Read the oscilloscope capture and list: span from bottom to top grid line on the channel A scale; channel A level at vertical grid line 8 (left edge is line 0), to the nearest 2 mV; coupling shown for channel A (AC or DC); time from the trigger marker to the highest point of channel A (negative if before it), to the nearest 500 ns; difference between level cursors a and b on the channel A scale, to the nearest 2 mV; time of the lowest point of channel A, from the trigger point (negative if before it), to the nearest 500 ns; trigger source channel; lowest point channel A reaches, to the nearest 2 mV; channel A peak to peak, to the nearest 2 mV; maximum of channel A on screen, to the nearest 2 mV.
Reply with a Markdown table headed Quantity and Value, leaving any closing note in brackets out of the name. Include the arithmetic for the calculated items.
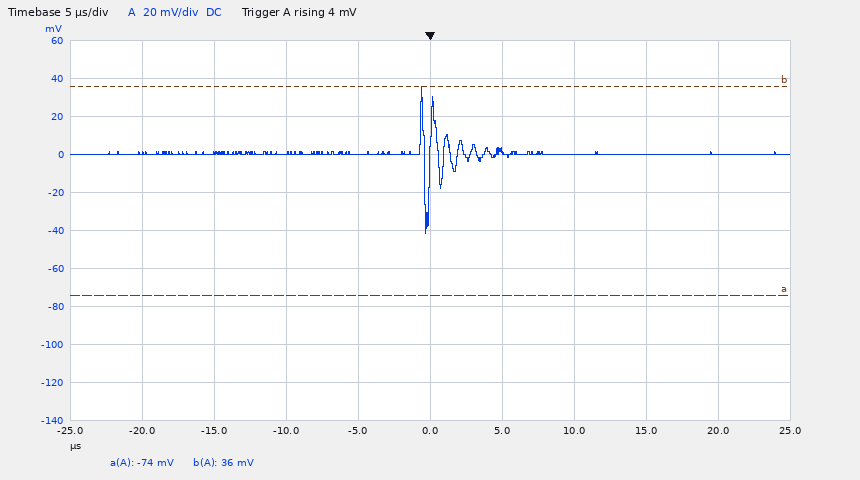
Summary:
| Quantity | Value |
|---|---|
| span from bottom to top grid line on the channel A scale | 200 mV |
| channel A level at vertical grid line 8 (left edge is line 0), to the nearest 2 mV | 0 mV |
| coupling shown for channel A | DC |
| time from the trigger marker to the highest point of channel A (negative if before it), to the nearest 500 ns | -500 ns |
| difference between level cursors a and b on the channel A scale, to the nearest 2 mV | 110 mV |
| time of the lowest point of channel A, from the trigger point (negative if before it), to the nearest 500 ns | -500 ns |
| trigger source channel | channel A |
| lowest point channel A reaches, to the nearest 2 mV | -42 mV |
| channel A peak to peak, to the nearest 2 mV | 36 mV − (-42 mV) = 78 mV |
| maximum of channel A on screen, to the nearest 2 mV | 36 mV |
